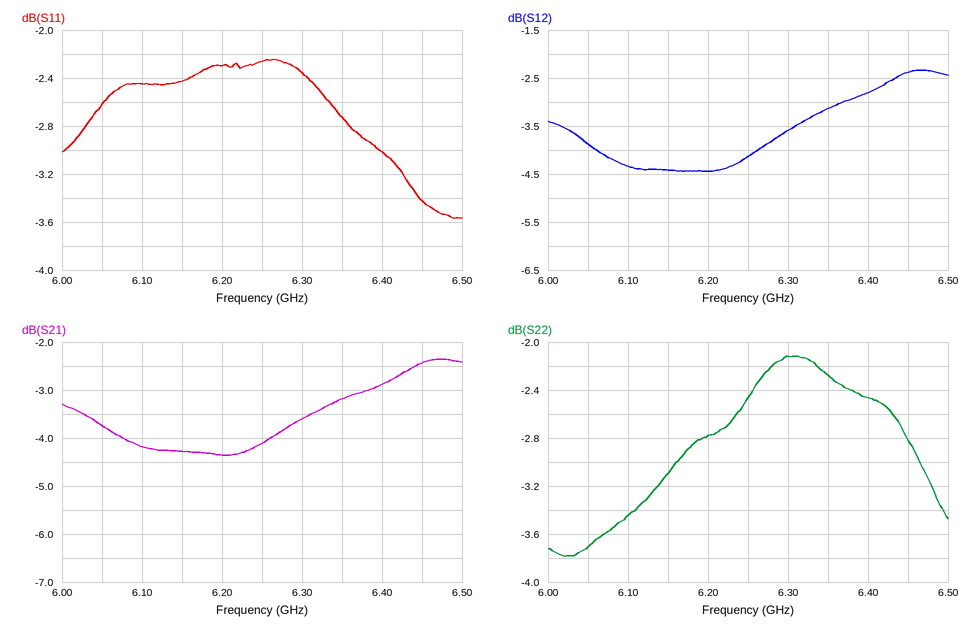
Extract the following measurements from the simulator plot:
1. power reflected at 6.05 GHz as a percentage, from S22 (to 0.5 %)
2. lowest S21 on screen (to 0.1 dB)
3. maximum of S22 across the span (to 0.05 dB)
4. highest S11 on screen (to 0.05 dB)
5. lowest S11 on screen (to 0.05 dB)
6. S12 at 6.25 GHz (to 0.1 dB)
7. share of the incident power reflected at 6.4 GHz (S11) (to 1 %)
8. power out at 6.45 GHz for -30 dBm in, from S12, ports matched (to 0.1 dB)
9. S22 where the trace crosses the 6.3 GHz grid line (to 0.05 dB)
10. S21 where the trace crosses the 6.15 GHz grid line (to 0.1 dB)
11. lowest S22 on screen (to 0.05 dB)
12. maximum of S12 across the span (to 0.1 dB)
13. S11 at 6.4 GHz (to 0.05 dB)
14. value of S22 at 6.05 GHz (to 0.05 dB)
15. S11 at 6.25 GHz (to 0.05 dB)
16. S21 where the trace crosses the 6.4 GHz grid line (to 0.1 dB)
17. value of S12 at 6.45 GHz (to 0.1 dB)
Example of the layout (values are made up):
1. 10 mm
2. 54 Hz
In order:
1. 42.5 %
2. -4.4 dB
3. -2.10 dB
4. -2.25 dB
5. -3.55 dB
6. -4.1 dB
7. 50 %
8. -32.4 dBm
9. -2.10 dB
10. -4.3 dB
11. -3.80 dB
12. -2.3 dB
13. -3.00 dB
14. -3.70 dB
15. -2.25 dB
16. -2.9 dB
17. -2.4 dB
